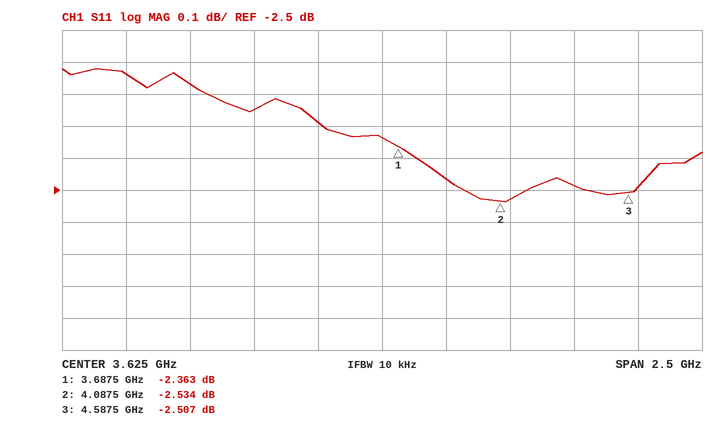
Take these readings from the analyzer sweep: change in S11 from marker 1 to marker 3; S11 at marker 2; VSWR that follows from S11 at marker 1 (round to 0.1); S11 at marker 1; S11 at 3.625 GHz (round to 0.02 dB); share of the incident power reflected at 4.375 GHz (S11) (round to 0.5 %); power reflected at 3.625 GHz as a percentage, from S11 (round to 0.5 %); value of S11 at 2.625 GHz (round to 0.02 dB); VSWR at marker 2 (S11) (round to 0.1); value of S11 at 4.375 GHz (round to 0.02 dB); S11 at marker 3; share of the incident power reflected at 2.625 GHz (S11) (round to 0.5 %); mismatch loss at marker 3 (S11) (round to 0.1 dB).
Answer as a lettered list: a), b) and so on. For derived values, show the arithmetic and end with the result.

a) -2.507 − (-2.363) = -0.144 dB
b) -2.534 dB
c) (1 + 0.7618)/(1 − 0.7618) ≈ 7.4
d) -2.363 dB
e) -2.34 dB
f) 10^(-2.48/10) ≈ 56.5 %
g) 10^(-2.34/10) ≈ 58.3 %, so 58.5 % to the nearest 0.5 %
h) -2.14 dB
i) (1 + 0.7470)/(1 − 0.7470) ≈ 6.9
j) -2.48 dB
k) -2.507 dB
l) 10^(-2.14/10) ≈ 61.1 %, so 61.0 % to the nearest 0.5 %
m) −10 log10(1 − 10^(-2.507/10)) ≈ 3.6 dB
